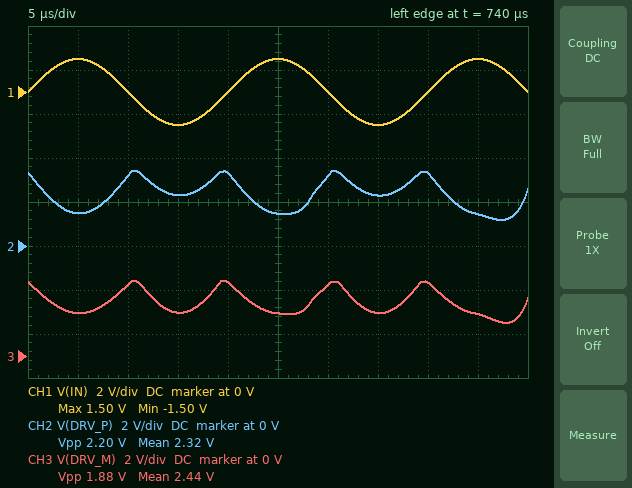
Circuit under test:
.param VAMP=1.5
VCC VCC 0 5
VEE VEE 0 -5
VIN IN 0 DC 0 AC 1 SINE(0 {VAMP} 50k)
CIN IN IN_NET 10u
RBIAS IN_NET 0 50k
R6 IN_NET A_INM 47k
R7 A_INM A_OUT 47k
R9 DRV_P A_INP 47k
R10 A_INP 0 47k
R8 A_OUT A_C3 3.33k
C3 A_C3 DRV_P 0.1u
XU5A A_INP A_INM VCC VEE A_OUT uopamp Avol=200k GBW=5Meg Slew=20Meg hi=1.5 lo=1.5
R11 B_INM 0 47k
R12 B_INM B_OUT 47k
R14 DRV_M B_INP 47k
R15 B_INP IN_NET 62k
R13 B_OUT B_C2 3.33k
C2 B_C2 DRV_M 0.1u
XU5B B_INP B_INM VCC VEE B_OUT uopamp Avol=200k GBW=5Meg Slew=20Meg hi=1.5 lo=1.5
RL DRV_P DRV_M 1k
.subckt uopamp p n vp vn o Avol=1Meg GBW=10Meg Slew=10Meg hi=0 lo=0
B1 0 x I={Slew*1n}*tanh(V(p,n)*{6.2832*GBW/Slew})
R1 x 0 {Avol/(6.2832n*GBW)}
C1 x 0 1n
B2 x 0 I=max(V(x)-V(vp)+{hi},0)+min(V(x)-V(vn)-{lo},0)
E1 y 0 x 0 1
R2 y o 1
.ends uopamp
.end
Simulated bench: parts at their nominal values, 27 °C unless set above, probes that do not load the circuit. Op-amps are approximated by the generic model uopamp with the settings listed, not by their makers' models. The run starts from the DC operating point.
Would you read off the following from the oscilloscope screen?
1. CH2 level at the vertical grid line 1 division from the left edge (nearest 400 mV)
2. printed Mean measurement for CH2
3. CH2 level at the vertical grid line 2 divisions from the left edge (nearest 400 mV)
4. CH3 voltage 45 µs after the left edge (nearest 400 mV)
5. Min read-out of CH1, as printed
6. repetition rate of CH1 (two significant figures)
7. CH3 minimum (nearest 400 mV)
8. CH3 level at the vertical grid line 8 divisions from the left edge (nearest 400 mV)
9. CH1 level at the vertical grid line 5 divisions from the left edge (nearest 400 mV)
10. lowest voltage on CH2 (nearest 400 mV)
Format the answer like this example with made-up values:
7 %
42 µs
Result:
1.6 V
2.32 V
3.2 V
2.0 V
-1.50 V
50 kHz
1.6 V
3.2 V
1.6 V
1.2 V
